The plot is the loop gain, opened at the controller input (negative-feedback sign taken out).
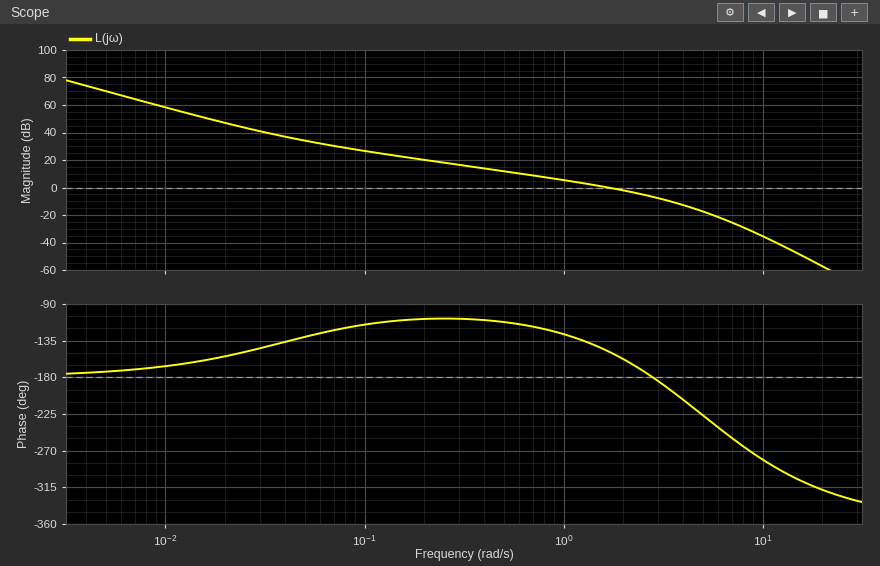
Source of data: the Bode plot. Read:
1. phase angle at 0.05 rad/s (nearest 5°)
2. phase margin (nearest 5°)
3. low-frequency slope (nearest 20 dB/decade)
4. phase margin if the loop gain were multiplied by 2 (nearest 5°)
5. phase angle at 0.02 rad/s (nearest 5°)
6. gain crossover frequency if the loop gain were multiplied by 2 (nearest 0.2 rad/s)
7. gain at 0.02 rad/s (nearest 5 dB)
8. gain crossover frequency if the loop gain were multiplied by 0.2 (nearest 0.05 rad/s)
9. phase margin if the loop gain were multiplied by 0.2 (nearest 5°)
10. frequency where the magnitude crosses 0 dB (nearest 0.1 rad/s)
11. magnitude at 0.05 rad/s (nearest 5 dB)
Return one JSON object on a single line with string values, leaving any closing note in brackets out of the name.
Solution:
{"phase angle at 0.05 rad/s": "-130°", "phase margin": "30°", "low-frequency slope": "-40 dB/decade", "phase margin if the loop gain were multiplied by 2": "5°", "phase angle at 0.02 rad/s": "-155°", "gain crossover frequency if the loop gain were multiplied by 2": "2.6 rad/s", "gain at 0.02 rad/s": "45 dB", "gain crossover frequency if the loop gain were multiplied by 0.2": "0.40 rad/s", "phase margin if the loop gain were multiplied by 0.2": "70°", "frequency where the magnitude crosses 0 dB": "1.7 rad/s", "magnitude at 0.05 rad/s": "35 dB"}
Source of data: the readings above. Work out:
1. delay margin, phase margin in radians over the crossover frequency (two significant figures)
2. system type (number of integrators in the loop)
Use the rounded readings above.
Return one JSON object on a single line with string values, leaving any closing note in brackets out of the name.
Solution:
{"delay margin, phase margin in radians over the crossover frequency": "0.31 s", "system type": "2"}
